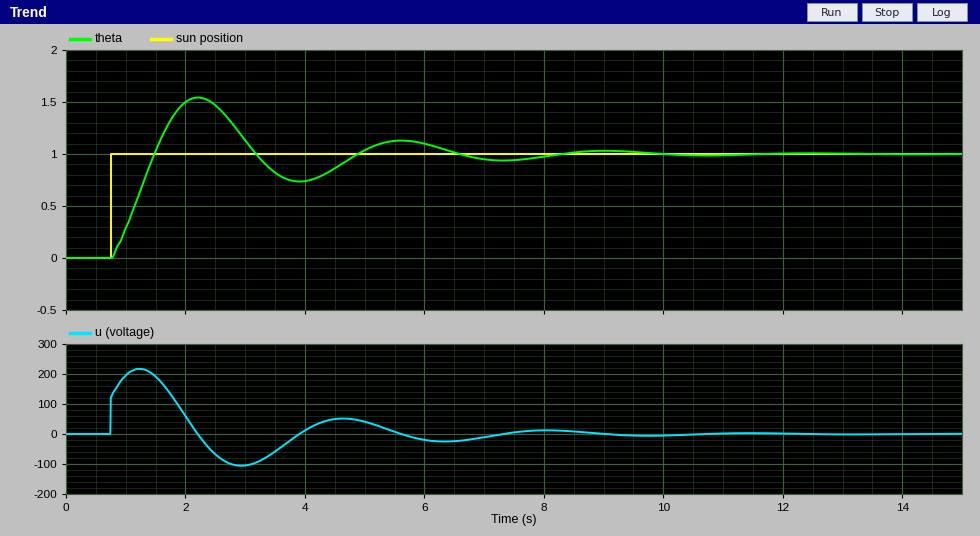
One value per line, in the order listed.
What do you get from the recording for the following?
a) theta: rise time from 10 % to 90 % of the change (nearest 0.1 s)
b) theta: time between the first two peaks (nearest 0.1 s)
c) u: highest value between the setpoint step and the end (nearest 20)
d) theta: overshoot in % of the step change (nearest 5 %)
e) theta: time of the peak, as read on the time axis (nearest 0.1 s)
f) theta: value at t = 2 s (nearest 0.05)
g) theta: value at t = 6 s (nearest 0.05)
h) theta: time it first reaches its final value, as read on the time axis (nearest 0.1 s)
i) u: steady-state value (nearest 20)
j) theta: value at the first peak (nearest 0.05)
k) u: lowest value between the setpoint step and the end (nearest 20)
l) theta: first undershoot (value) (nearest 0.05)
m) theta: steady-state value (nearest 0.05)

0.6 s
3.4 s
220
55 %
2.2 s
1.50
1.10
1.5 s
0
1.55
-100
0.75
1.00
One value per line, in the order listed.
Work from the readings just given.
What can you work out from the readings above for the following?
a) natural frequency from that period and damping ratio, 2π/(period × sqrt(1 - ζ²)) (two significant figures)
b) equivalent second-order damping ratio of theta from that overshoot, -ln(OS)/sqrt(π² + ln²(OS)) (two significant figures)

1.9 rad/s
0.19
